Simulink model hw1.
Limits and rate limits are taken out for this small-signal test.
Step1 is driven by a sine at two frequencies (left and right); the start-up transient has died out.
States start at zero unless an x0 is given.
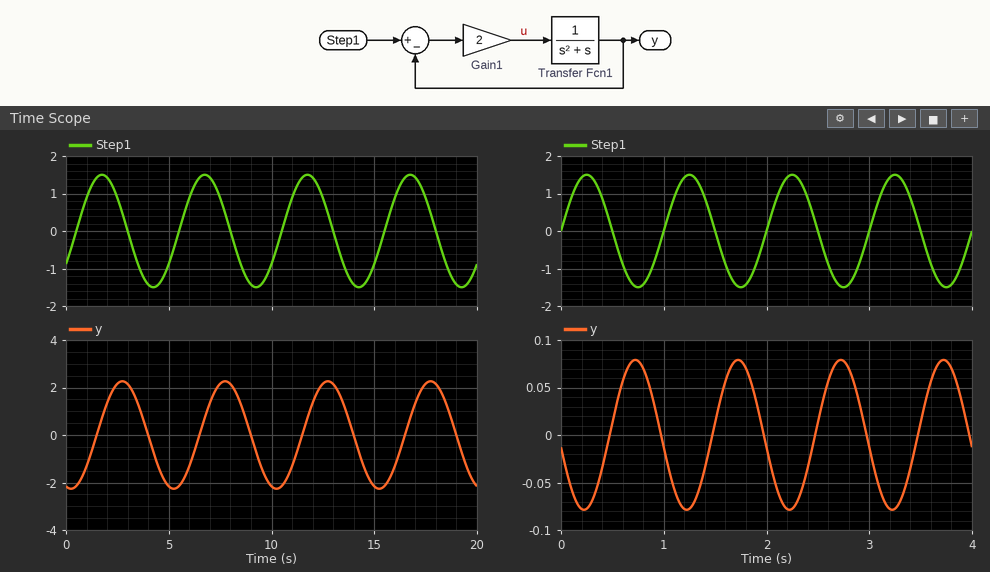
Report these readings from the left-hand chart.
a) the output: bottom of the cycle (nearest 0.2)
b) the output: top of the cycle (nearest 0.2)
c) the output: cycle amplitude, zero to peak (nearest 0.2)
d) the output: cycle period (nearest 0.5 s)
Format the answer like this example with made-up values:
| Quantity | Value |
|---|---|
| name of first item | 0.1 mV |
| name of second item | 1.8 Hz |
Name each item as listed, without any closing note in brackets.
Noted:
| Quantity | Value |
|---|---|
| the output: bottom of the cycle | -2.2 |
| the output: top of the cycle | 2.2 |
| the output: cycle amplitude, zero to peak | 2.2 |
| the output: cycle period | 5.0 s |
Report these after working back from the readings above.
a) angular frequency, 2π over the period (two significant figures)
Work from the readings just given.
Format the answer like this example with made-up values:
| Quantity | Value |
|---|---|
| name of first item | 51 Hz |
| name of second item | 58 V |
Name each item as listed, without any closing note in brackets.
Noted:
| Quantity | Value |
|---|---|
| angular frequency, 2π over the period | 1.3 rad/s |
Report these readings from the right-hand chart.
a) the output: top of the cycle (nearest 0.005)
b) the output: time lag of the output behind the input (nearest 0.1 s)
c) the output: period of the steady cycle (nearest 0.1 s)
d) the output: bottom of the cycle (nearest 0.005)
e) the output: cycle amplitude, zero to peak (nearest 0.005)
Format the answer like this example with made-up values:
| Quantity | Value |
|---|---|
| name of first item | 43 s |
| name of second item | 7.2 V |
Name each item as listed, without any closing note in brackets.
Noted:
| Quantity | Value |
|---|---|
| the output: top of the cycle | 0.080 |
| the output: time lag of the output behind the input | 0.5 s |
| the output: period of the steady cycle | 1.0 s |
| the output: bottom of the cycle | -0.080 |
| the output: cycle amplitude, zero to peak | 0.080 |
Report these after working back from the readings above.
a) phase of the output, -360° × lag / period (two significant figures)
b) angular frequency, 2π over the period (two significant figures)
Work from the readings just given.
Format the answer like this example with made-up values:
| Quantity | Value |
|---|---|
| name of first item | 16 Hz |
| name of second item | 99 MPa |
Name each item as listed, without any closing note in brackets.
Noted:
| Quantity | Value |
|---|---|
| phase of the output, -360° × lag / period | -180° |
| angular frequency, 2π over the period | 6.3 rad/s |
